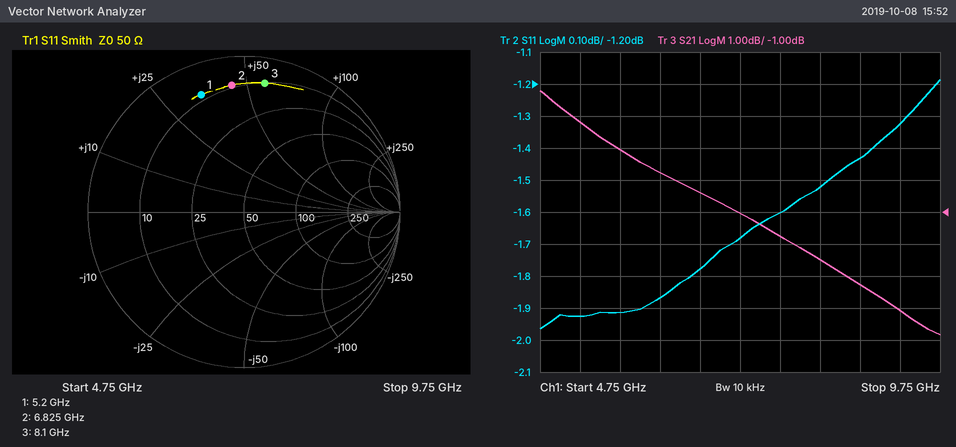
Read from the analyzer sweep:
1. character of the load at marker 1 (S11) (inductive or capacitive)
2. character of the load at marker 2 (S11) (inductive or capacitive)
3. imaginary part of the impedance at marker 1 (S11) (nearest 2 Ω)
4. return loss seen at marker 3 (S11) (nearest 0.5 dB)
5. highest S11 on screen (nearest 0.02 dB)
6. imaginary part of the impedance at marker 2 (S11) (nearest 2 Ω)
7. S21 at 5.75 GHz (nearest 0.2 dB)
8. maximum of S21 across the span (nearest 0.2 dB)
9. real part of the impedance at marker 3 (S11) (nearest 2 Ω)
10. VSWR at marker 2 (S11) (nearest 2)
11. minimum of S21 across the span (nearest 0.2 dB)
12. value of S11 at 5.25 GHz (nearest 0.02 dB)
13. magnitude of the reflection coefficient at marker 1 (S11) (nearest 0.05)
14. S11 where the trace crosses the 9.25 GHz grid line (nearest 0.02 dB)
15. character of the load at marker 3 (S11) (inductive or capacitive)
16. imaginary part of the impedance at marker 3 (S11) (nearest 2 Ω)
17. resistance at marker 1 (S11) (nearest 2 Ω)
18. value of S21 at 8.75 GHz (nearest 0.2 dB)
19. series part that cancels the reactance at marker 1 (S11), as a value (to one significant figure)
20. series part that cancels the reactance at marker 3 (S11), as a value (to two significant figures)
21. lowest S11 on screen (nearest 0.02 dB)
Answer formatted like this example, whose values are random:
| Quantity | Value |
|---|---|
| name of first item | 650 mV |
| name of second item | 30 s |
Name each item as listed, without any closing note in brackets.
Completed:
| Quantity | Value |
|---|---|
| character of the load at marker 1 (S11) | inductive |
| character of the load at marker 2 (S11) | inductive |
| imaginary part of the impedance at marker 1 (S11) | +34 Ω |
| return loss seen at marker 3 (S11) | 1.5 dB |
| highest S11 on screen | -1.18 dB |
| imaginary part of the impedance at marker 2 (S11) | +44 Ω |
| S21 at 5.75 GHz | 1.0 dB |
| maximum of S21 across the span | 2.8 dB |
| real part of the impedance at marker 3 (S11) | 10 Ω |
| VSWR at marker 2 (S11) | 10 |
| minimum of S21 across the span | -4.8 dB |
| value of S11 at 5.25 GHz | -1.92 dB |
| magnitude of the reflection coefficient at marker 1 (S11) | 0.80 |
| S11 where the trace crosses the 9.25 GHz grid line | -1.32 dB |
| character of the load at marker 3 (S11) | inductive |
| imaginary part of the impedance at marker 3 (S11) | +58 Ω |
| resistance at marker 1 (S11) | 8 Ω |
| value of S21 at 8.75 GHz | -3.2 dB |
| series part that cancels the reactance at marker 1 (S11), as a value | 900 fF |
| series part that cancels the reactance at marker 3 (S11), as a value | 340 fF |
| lowest S11 on screen | -1.96 dB |
